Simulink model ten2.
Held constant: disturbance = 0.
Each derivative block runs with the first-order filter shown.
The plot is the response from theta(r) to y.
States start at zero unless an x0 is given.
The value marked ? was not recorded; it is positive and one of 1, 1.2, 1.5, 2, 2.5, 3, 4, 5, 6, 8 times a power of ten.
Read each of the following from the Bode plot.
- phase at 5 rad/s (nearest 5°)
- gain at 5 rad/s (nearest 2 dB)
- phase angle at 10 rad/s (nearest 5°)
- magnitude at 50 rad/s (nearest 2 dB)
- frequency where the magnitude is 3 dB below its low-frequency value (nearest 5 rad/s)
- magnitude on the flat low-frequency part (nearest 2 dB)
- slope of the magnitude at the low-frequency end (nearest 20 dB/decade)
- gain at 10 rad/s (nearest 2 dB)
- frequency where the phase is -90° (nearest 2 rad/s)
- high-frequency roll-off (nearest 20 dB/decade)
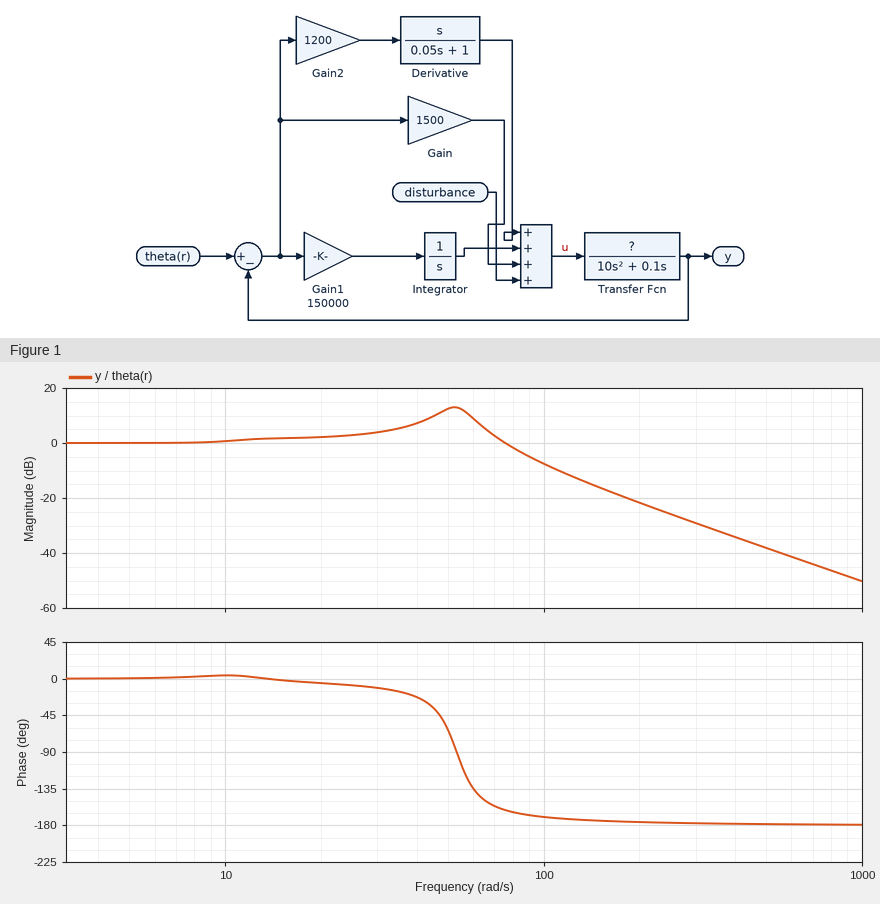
0°
0 dB
5°
12 dB
85 rad/s
0 dB
0 dB/decade
0 dB
54 rad/s
-40 dB/decade
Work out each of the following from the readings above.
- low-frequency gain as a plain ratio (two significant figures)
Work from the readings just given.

1.0
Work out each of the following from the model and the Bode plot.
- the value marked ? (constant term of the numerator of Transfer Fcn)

1.2
